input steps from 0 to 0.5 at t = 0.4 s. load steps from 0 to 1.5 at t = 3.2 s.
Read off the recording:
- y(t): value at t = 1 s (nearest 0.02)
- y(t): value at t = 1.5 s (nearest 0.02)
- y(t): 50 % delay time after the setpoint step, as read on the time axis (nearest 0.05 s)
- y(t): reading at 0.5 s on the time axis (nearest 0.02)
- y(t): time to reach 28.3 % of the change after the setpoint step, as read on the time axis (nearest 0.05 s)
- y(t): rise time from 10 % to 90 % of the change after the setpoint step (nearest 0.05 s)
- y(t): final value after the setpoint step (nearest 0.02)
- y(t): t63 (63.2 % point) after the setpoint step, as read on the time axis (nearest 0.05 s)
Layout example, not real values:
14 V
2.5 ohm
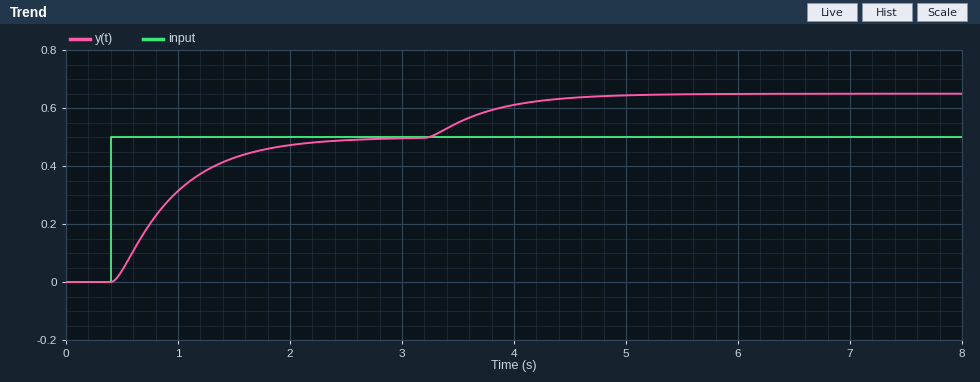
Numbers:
0.32
0.42
0.85 s
0.04
0.65 s
1.15 s
0.50
1.00 s
